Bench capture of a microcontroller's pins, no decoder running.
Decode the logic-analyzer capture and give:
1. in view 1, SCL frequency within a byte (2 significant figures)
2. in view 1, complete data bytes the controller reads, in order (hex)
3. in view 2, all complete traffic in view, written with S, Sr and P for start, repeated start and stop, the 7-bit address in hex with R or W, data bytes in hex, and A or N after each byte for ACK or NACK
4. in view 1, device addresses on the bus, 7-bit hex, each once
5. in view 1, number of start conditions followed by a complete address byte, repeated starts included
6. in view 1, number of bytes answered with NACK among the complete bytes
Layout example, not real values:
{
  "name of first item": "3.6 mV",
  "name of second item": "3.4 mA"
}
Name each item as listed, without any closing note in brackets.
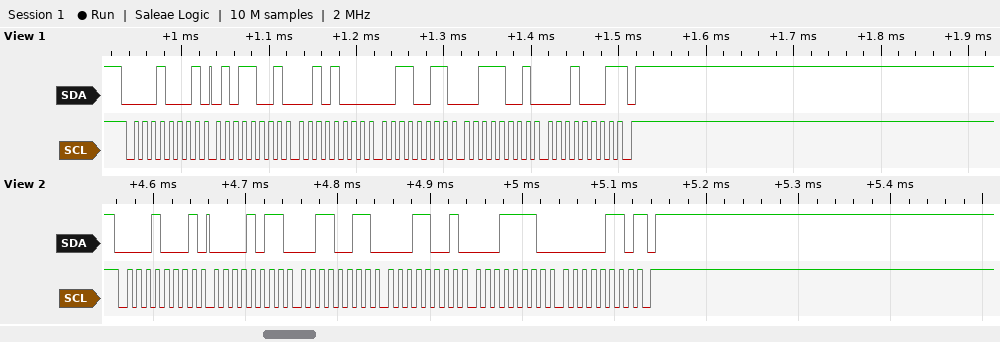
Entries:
{
  "in view 1, SCL frequency within a byte": "100 kHz",
  "in view 1, complete data bytes the controller reads, in order": "59 28 33 39 11",
  "in view 2, all complete traffic in view, written with S, Sr and P for start, repeated start and stop, the 7-bit address in hex with R or W, data bytes in hex, and A or N after each byte for ACK or NACK": "S 08R A 0B A 33 A 19 A 1E A 06 N P",
  "in view 1, device addresses on the bus, 7-bit hex, each once": "0x08",
  "in view 1, number of start conditions followed by a complete address byte, repeated starts included": "1",
  "in view 1, number of bytes answered with NACK among the complete bytes": "1"
}
